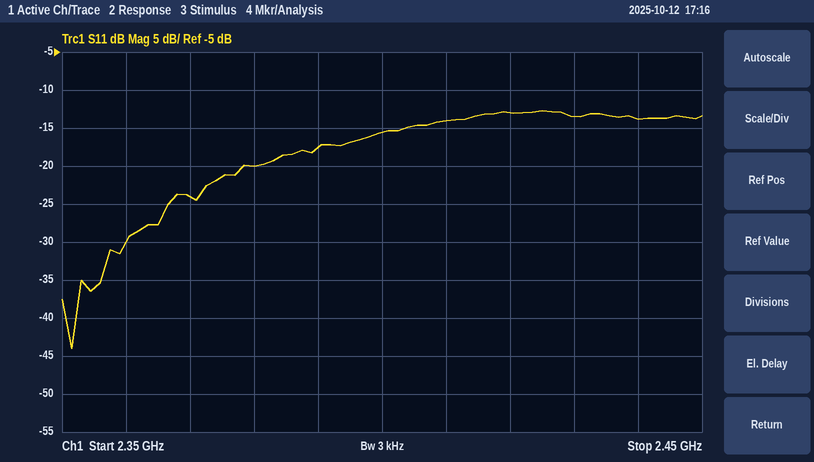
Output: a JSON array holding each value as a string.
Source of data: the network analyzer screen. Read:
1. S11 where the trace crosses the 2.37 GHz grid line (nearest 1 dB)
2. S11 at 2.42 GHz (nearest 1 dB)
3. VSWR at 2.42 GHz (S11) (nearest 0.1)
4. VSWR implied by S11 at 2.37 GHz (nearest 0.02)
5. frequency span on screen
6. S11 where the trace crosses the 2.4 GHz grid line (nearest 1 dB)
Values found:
["-24 dB", "-13 dB", "1.6", "1.14", "100 MHz", "-16 dB"]
